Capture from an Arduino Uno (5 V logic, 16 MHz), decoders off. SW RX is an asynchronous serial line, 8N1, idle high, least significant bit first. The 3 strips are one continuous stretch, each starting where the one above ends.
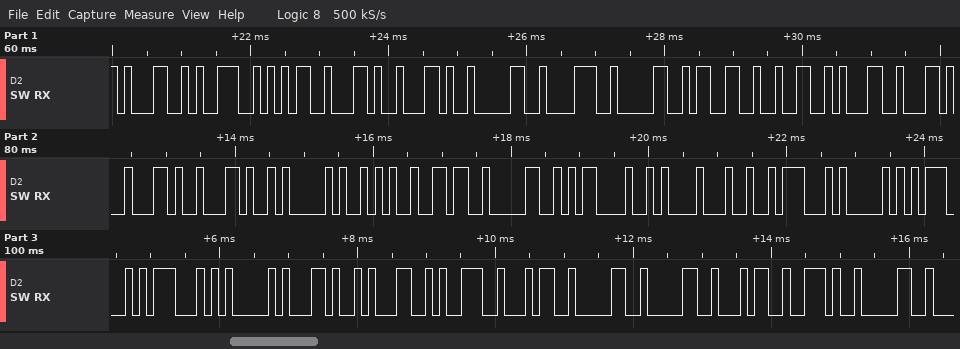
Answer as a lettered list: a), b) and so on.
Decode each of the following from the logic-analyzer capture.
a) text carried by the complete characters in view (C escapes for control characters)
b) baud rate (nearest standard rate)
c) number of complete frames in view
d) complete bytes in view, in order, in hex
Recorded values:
a) "195,,080321,,,A*60\r\n$GPGGA,194004.0"
b) 9600 baud
c) 35
d) 31 39 35 2C 2C 30 38 30 33 32 31 2C 2C 2C 41 2A 36 30 0D 0A 24 47 50 47 47 41 2C 31 39 34 30 30 34 2E 30
